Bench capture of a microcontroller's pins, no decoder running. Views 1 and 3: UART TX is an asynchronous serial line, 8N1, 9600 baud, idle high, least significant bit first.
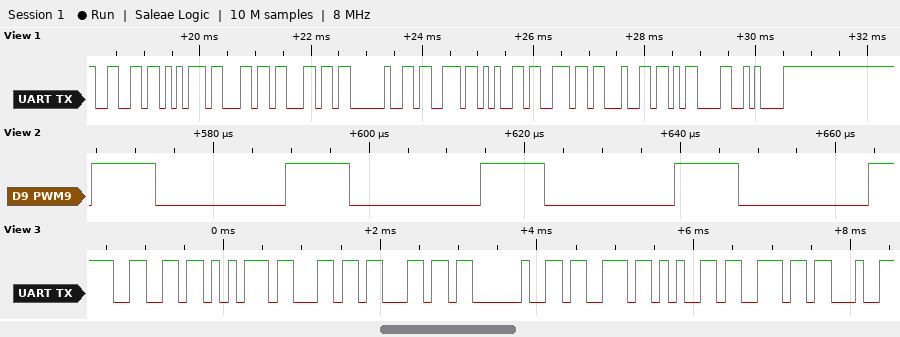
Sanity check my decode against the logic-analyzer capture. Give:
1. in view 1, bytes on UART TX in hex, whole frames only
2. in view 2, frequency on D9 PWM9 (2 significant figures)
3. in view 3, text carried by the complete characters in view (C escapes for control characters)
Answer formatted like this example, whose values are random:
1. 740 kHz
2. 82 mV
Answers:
1. 0x66 0x75 0x6C 0x6C 0x20 0x73 0x65 0x6E 0x64 0x0D 0x0A
2. 40 kHz
3. "full sen"
